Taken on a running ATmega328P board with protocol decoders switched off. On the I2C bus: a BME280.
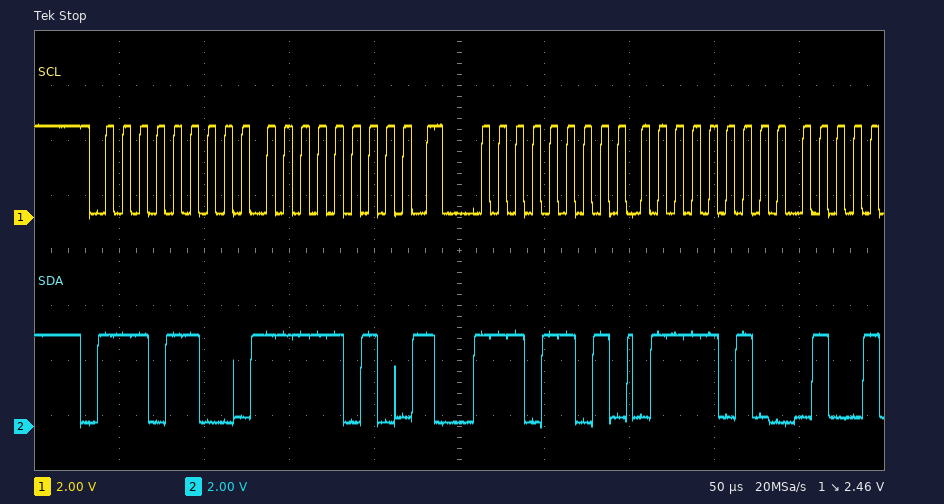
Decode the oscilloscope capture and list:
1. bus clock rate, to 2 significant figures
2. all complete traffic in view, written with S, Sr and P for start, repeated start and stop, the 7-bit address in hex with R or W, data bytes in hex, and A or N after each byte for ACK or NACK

100 kHz
S 76W A FA A Sr 76R A 7A A
